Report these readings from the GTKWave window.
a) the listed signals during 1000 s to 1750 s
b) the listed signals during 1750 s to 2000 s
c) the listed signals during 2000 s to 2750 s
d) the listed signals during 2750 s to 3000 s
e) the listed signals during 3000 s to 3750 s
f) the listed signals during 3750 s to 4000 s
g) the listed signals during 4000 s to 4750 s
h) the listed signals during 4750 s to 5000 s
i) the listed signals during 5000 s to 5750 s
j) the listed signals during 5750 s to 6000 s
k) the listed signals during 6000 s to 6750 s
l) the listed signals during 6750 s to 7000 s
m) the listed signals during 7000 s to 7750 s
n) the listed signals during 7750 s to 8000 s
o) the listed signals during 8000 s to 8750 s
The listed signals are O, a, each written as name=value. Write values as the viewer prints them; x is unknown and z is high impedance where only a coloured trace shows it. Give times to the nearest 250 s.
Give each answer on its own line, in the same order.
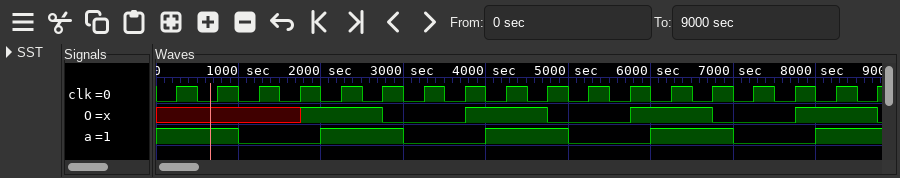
O=x, a=0
O=1, a=0
O=1, a=1
O=0, a=1
O=0, a=0
O=1, a=0
O=1, a=1
O=0, a=1
O=0, a=0
O=1, a=0
O=1, a=1
O=0, a=1
O=0, a=0
O=1, a=0
O=1, a=1
